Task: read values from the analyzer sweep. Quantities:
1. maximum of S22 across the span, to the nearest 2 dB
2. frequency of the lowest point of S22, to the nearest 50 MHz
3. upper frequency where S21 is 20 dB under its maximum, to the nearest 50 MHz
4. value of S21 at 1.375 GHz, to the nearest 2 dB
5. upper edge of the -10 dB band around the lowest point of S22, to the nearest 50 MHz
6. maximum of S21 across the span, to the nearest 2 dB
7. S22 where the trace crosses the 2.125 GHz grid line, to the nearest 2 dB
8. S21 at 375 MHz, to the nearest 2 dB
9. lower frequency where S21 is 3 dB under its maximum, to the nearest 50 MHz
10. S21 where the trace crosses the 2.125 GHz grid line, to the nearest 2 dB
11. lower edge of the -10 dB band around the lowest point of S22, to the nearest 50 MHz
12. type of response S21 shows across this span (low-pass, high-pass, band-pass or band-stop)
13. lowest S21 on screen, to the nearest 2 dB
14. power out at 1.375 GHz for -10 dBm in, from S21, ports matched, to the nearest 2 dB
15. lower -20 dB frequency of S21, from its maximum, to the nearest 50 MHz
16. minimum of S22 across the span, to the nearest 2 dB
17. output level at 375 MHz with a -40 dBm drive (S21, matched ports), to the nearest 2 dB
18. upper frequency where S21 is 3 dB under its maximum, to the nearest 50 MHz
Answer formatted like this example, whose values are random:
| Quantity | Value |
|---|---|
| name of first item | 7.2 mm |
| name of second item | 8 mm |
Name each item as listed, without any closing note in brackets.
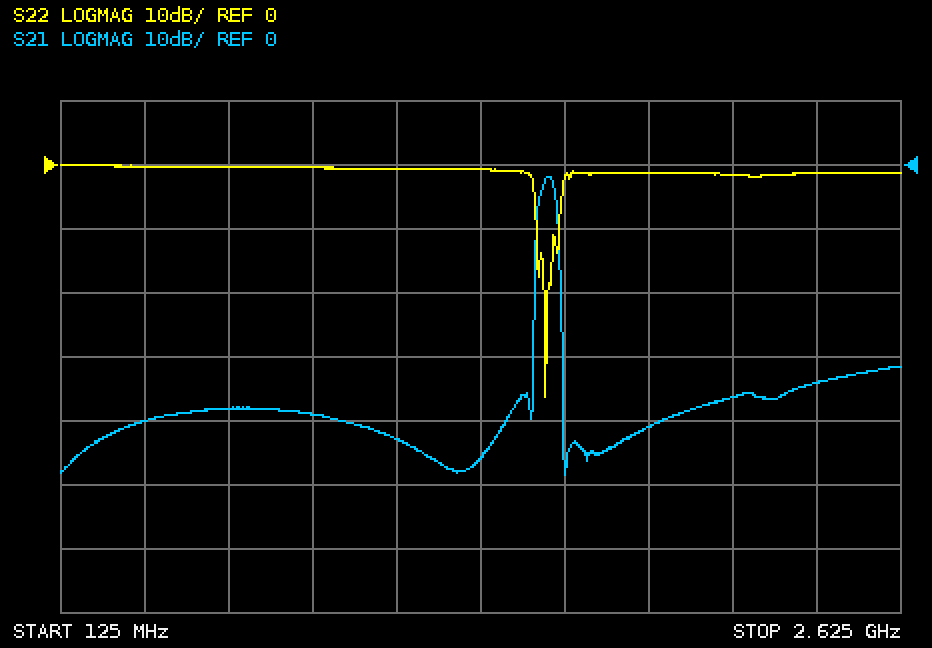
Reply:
| Quantity | Value |
|---|---|
| maximum of S22 across the span, to the nearest 2 dB | 0 dB |
| frequency of the lowest point of S22, to the nearest 50 MHz | 1.55 GHz |
| upper frequency where S21 is 20 dB under its maximum, to the nearest 50 MHz | 1.60 GHz |
| value of S21 at 1.375 GHz, to the nearest 2 dB | -46 dB |
| upper edge of the -10 dB band around the lowest point of S22, to the nearest 50 MHz | 1.60 GHz |
| maximum of S21 across the span, to the nearest 2 dB | -2 dB |
| S22 where the trace crosses the 2.125 GHz grid line, to the nearest 2 dB | -2 dB |
| S21 at 375 MHz, to the nearest 2 dB | -40 dB |
| lower frequency where S21 is 3 dB under its maximum, to the nearest 50 MHz | 1.55 GHz |
| S21 where the trace crosses the 2.125 GHz grid line, to the nearest 2 dB | -36 dB |
| lower edge of the -10 dB band around the lowest point of S22, to the nearest 50 MHz | 1.55 GHz |
| type of response S21 shows across this span | band-pass |
| lowest S21 on screen, to the nearest 2 dB | -48 dB |
| power out at 1.375 GHz for -10 dBm in, from S21, ports matched, to the nearest 2 dB | -56 dBm |
| lower -20 dB frequency of S21, from its maximum, to the nearest 50 MHz | 1.55 GHz |
| minimum of S22 across the span, to the nearest 2 dB | -36 dB |
| output level at 375 MHz with a -40 dBm drive (S21, matched ports), to the nearest 2 dB | -80 dBm |
| upper frequency where S21 is 3 dB under its maximum, to the nearest 50 MHz | 1.60 GHz |
